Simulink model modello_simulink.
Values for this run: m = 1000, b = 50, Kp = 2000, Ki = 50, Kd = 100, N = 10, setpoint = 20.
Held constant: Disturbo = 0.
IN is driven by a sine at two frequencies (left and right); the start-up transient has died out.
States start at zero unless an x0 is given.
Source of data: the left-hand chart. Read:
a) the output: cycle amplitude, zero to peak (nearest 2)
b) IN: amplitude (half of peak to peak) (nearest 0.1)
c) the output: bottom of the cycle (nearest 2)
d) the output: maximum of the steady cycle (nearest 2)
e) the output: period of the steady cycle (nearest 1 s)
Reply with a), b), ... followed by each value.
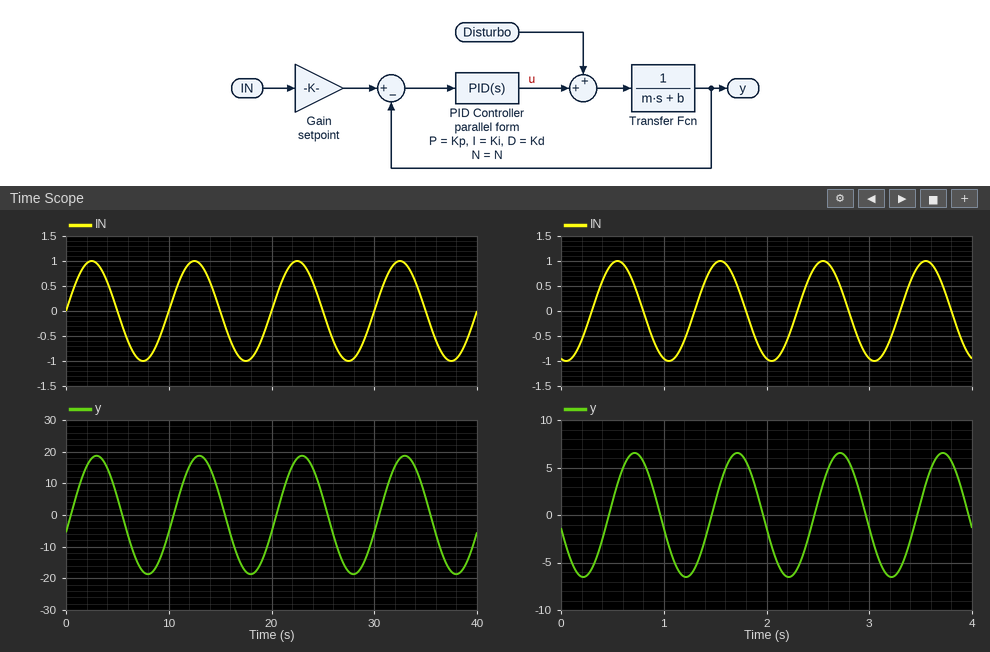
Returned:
a) 18
b) 1.0
c) -18
d) 18
e) 10 s
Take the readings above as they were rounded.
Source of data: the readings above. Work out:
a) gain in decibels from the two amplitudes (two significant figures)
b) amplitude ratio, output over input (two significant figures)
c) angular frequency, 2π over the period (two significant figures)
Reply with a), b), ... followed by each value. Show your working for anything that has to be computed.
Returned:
a) 20 log10(18 / 1) = 25 dB
b) 18 / 1 = 18
c) 2π / 10 = 0.63 rad/s
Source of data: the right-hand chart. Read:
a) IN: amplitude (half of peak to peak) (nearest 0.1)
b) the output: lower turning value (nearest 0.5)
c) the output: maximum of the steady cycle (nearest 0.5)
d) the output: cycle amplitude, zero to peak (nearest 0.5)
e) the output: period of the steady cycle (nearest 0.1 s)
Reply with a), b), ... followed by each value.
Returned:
a) 1.0
b) -6.5
c) 6.5
d) 6.5
e) 1.0 s
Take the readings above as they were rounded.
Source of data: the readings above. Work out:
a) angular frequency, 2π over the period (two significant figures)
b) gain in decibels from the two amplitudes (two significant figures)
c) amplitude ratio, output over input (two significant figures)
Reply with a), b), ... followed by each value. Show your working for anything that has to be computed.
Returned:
a) 2π / 1 = 6.3 rad/s
b) 20 log10(6.5 / 1) = 16 dB
c) 6.5 / 1 = 6.5
